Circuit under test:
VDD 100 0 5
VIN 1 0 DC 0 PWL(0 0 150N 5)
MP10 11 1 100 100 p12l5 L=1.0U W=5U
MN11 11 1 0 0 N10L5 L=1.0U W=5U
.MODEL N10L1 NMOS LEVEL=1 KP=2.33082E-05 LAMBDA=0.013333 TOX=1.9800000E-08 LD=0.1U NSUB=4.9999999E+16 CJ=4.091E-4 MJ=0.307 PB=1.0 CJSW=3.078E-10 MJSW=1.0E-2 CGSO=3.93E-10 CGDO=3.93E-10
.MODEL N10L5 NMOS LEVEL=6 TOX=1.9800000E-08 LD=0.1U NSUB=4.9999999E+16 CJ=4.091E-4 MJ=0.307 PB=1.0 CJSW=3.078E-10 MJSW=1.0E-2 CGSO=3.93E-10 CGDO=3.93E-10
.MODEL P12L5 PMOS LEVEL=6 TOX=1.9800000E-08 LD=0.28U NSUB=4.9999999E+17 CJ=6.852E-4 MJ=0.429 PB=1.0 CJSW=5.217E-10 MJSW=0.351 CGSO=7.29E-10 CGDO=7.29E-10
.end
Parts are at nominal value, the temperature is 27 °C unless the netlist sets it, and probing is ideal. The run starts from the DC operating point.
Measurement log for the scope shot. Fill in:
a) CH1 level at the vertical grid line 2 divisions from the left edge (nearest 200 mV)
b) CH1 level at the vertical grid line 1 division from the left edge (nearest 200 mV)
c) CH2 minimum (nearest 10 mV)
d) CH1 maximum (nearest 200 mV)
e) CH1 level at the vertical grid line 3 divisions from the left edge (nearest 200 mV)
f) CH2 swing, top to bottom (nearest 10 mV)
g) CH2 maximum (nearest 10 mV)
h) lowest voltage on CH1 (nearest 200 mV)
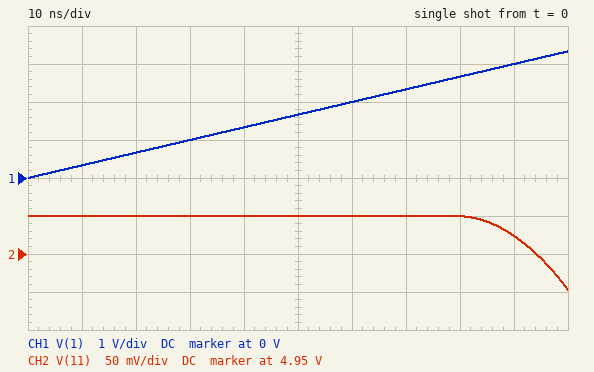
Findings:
600 mV
400 mV
4.90 V
3.4 V
1.0 V
100 mV
5.00 V
0 V
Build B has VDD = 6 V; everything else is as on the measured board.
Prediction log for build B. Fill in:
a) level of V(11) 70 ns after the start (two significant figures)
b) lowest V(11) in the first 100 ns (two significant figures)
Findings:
6.0 V
5.9 V
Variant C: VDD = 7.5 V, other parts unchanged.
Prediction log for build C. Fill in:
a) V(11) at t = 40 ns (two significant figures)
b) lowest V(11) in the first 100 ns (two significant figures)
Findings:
7.5 V
7.4 V
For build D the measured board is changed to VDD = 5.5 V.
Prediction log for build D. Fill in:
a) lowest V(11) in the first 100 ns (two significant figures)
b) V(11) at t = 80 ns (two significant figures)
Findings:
5.4 V
5.5 V
